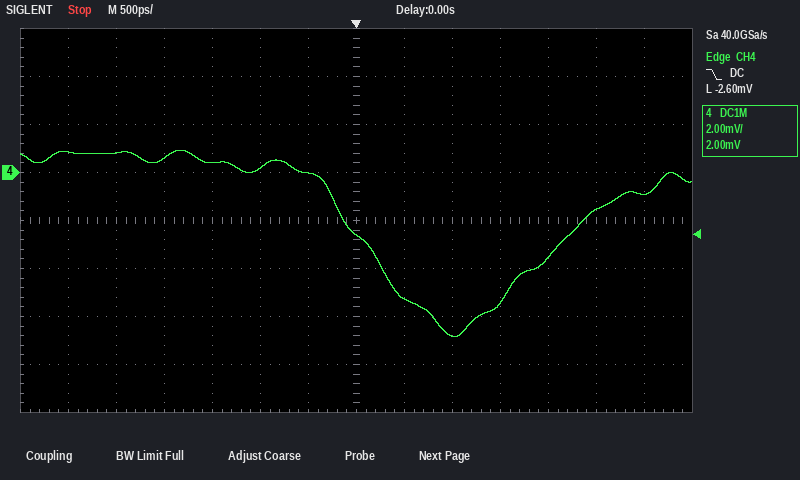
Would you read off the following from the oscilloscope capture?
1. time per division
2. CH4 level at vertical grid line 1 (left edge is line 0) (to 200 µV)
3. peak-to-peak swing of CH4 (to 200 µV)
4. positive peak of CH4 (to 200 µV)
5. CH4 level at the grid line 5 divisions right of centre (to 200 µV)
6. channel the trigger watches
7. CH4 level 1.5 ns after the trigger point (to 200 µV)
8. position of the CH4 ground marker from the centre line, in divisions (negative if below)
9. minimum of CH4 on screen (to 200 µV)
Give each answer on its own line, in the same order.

500 ps
800 µV
7.8 mV
1.0 mV
-1.6 mV
CH4
-5.4 mV
+1.0 div
-6.8 mV
